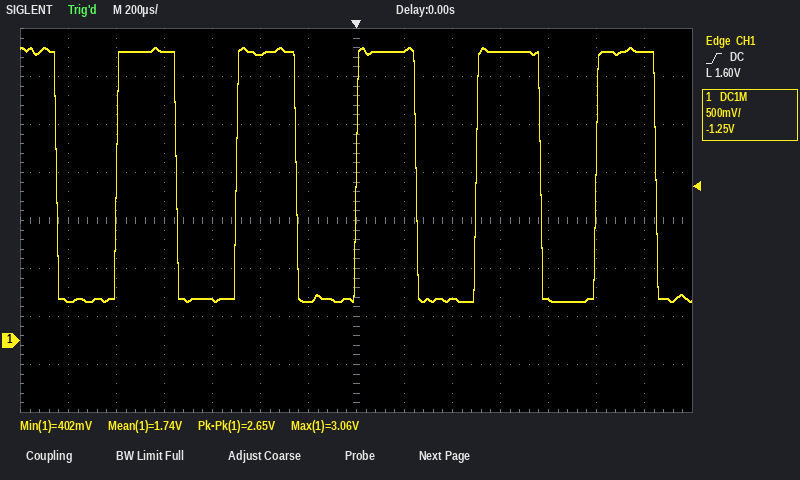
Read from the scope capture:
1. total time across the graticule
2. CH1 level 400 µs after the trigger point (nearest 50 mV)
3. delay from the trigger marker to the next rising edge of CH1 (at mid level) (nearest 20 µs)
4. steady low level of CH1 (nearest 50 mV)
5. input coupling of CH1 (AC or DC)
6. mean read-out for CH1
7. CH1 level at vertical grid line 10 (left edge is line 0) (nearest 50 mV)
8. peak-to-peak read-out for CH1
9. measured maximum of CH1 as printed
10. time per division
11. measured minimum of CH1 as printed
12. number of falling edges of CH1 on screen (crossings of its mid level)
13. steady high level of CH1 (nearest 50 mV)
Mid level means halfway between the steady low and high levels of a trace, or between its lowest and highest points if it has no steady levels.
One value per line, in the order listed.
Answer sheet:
2.8 ms
450 mV
500 µs
450 mV
DC
1.74 V
3.00 V
2.65 V
3.06 V
200 µs
402 mV
6
3.00 V
